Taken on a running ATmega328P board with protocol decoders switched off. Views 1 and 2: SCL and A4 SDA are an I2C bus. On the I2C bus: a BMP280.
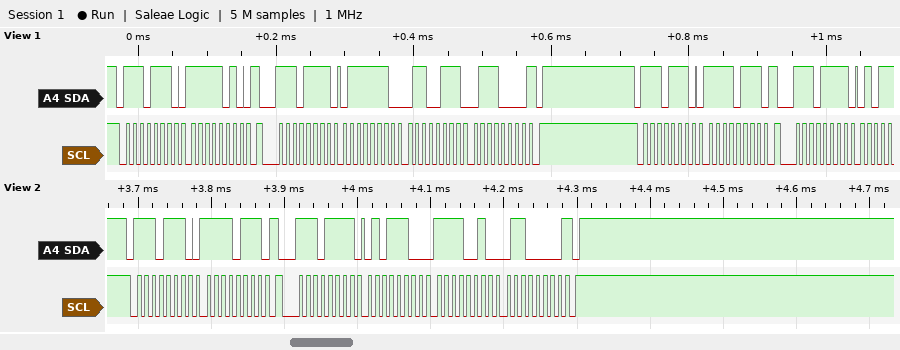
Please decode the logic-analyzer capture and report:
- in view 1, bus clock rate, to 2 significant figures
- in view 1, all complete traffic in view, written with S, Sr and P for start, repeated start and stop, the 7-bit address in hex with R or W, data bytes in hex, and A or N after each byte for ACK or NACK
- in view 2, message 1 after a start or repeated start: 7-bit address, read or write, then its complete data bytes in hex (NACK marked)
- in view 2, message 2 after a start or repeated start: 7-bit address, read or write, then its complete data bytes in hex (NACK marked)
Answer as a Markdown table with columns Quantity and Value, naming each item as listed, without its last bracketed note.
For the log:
| Quantity | Value |
|---|---|
| in view 1, bus clock rate, to 2 significant figures | 100 kHz |
| in view 1, all complete traffic in view, written with S, Sr and P for start, repeated start and stop, the 7-bit address in hex with R or W, data bytes in hex, and A or N after each byte for ACK or NACK | S 77W A FA A Sr 77R A 7E A 67 A 70 N P S 77W A F7 A Sr 77R A |
| in view 2, message 1 after a start or repeated start: 7-bit address, read or write, then its complete data bytes in hex | 0x77 write: F7 |
| in view 2, message 2 after a start or repeated start: 7-bit address, read or write, then its complete data bytes in hex | 0x77 read: 5C F2 60 NACK |
